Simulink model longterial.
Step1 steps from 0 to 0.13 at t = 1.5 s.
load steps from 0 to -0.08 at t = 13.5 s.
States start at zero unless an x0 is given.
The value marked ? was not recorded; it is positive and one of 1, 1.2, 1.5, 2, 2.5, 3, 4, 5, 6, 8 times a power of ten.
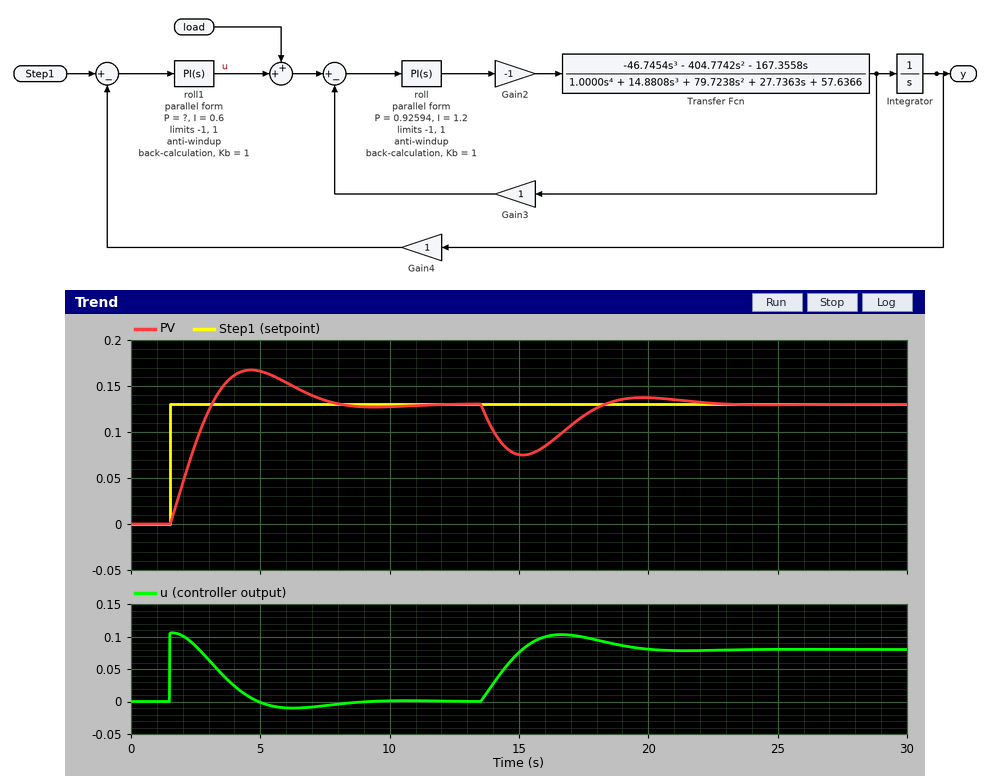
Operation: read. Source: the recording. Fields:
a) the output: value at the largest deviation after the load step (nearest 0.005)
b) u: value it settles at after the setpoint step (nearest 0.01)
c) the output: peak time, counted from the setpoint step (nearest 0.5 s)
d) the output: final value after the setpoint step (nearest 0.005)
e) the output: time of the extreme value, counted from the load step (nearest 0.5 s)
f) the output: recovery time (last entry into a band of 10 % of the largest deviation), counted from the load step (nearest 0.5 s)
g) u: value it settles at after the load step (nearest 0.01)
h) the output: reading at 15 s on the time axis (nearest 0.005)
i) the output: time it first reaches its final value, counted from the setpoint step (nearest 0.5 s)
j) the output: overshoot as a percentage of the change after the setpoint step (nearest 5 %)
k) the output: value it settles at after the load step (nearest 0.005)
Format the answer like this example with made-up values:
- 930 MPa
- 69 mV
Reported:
- 0.075
- 0.00
- 3.0 s
- 0.130
- 1.5 s
- 7.5 s
- 0.08
- 0.075
- 1.5 s
- 30 %
- 0.130
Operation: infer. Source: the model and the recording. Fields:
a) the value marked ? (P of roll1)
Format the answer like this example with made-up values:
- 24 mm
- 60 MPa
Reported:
- 0.8
